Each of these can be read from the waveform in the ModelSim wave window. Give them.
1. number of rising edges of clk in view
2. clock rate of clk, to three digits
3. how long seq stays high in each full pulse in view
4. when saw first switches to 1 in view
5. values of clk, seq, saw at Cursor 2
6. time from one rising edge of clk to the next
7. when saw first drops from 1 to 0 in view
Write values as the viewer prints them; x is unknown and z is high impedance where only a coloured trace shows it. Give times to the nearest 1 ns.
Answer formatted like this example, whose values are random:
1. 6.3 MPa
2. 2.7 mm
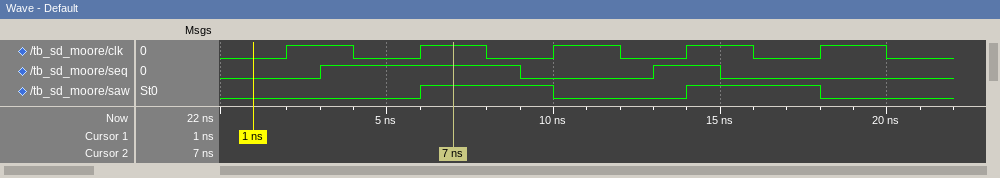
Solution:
1. 5
2. 250 MHz
3. 6 ns, 2 ns
4. 6 ns
5. clk=1, seq=1, saw=1
6. 4 ns
7. 10 ns
